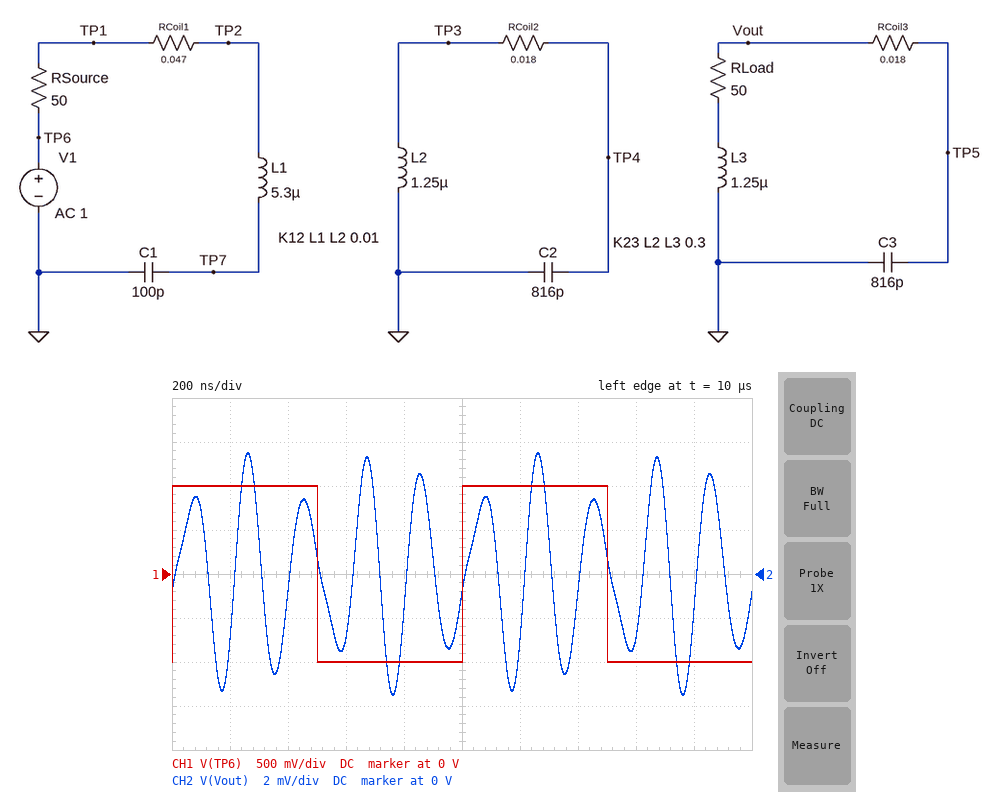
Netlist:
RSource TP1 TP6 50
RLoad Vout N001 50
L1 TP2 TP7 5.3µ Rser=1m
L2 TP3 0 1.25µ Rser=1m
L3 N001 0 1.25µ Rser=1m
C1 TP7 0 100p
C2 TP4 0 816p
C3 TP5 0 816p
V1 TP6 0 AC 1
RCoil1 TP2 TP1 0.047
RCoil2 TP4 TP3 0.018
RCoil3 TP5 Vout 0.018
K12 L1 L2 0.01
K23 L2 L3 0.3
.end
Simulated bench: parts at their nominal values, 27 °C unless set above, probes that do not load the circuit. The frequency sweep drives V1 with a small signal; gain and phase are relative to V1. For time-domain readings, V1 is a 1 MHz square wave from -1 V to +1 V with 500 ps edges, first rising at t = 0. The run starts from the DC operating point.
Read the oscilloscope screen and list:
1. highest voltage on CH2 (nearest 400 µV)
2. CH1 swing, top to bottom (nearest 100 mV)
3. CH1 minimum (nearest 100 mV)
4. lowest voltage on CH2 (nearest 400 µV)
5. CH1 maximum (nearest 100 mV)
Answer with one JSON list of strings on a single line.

["5.6 mV", "2.0 V", "-1.0 V", "-5.6 mV", "1.0 V"]
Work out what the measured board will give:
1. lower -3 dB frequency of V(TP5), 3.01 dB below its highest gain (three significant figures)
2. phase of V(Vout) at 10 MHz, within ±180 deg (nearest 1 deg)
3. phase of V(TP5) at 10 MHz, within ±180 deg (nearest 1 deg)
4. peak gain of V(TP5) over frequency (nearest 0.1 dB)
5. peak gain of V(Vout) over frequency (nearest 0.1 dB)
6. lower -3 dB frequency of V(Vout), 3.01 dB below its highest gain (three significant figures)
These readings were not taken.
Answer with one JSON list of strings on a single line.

["4.83 MHz", "61 deg", "61 deg", "-35.6 dB", "-35.6 dB", "4.83 MHz"]
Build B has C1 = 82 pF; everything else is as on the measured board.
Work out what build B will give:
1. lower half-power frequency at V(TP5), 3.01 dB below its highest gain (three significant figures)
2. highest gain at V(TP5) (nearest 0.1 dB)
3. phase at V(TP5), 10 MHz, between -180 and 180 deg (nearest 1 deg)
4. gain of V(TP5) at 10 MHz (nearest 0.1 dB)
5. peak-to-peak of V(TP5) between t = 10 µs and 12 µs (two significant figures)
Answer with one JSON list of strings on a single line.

["4.83 MHz", "-38.7 dB", "65 deg", "-58.3 dB", "8.5 mV"]
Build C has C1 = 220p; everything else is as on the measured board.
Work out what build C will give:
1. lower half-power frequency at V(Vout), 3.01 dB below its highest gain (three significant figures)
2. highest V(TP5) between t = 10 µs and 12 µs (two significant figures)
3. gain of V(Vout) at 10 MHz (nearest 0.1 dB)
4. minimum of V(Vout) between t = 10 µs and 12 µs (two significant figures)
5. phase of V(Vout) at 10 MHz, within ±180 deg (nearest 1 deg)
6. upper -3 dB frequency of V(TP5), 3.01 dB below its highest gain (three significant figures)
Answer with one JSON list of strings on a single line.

["4.78 MHz", "13 mV", "-63.4 dB", "-13 mV", "56 deg", "5.14 MHz"]
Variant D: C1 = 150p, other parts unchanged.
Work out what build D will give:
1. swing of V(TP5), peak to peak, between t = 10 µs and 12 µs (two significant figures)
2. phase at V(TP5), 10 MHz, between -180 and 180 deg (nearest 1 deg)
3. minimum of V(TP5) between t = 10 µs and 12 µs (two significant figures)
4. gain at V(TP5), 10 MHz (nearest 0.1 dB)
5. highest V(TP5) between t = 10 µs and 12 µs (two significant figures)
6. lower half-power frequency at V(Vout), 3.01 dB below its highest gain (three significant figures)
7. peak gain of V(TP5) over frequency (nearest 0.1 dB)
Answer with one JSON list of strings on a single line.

["21 mV", "58 deg", "-11 mV", "-62.3 dB", "11 mV", "4.84 MHz", "-28.2 dB"]
